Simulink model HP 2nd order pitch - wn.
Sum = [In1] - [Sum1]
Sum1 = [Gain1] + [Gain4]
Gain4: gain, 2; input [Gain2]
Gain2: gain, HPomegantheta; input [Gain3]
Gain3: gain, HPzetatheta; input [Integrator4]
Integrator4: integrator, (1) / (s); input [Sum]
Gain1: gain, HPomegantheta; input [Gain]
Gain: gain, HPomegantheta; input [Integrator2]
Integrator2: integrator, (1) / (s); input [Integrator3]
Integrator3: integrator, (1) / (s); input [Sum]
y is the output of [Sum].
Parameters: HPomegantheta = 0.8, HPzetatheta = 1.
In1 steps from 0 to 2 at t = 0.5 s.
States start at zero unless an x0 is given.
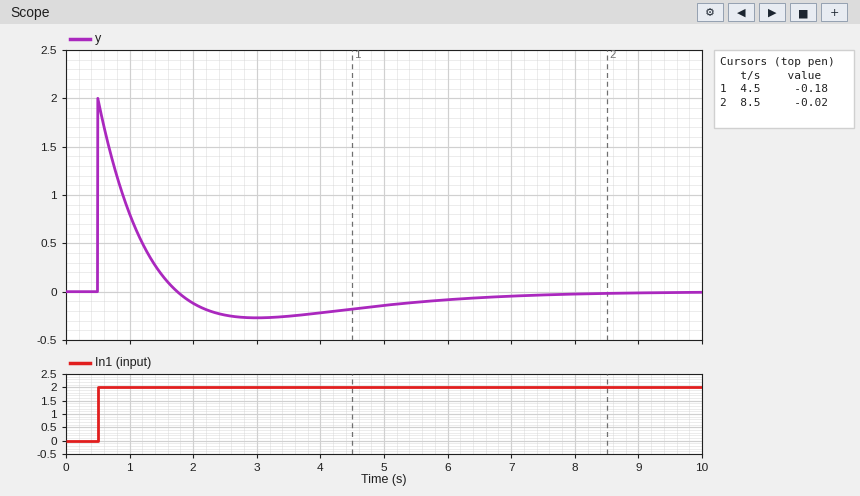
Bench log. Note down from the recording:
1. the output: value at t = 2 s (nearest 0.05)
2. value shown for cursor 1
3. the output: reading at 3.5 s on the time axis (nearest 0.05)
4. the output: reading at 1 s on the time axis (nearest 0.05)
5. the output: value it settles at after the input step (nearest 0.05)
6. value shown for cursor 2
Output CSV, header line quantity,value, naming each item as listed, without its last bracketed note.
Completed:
quantity,value
the output: value at t = 2 s,-0.10
value shown for cursor 1,-0.18
the output: reading at 3.5 s on the time axis,-0.25
the output: reading at 1 s on the time axis,0.80
the output: value it settles at after the input step,0.00
value shown for cursor 2,-0.02
